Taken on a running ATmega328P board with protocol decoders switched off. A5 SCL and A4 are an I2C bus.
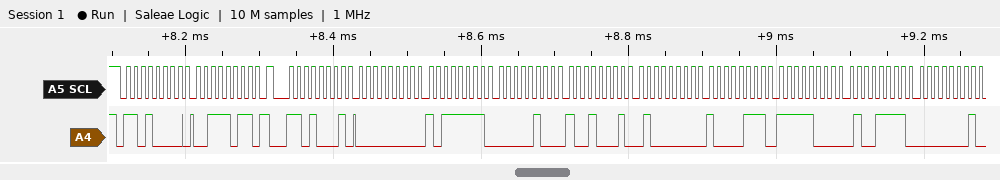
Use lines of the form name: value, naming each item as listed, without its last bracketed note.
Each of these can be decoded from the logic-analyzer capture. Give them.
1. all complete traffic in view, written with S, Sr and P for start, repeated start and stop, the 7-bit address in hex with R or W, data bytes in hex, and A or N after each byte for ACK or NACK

all complete traffic in view, written with S, Sr and P for start, repeated start and stop, the 7-bit address in hex with R or W, data bytes in hex, and A or N after each byte for ACK or NACK: S 68W A 3B A Sr 68R A 00 A BF A 04 A 91 A 40 A 87 A F8 A 4F A 01 A
